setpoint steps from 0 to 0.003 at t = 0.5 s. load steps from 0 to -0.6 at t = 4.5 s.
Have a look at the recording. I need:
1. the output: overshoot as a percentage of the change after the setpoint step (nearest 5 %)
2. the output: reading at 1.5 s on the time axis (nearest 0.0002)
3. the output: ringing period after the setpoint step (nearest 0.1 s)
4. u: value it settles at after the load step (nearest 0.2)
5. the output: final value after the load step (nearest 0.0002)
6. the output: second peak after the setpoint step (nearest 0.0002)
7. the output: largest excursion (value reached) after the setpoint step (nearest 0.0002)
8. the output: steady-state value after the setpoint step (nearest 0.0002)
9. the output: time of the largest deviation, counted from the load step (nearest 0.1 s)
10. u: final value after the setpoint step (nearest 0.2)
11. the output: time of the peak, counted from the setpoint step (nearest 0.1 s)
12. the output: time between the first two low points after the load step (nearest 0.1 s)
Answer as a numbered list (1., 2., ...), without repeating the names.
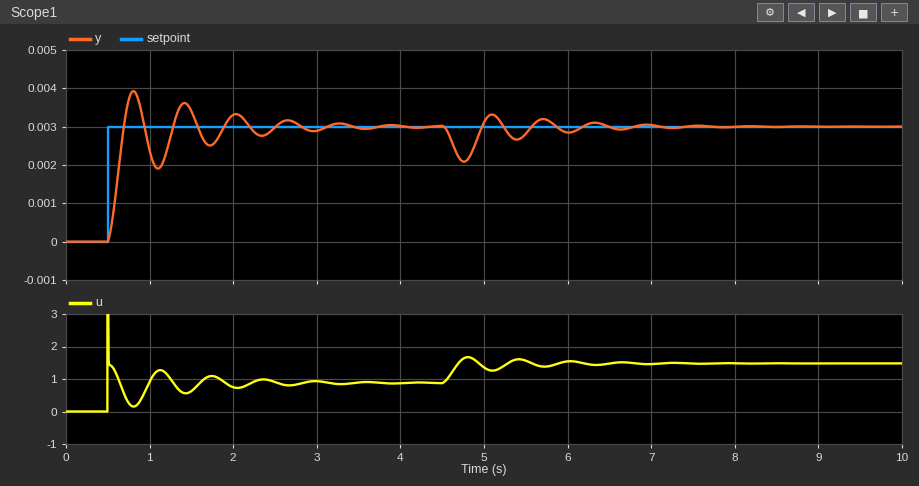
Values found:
1. 30 %
2. 0.0034
3. 0.6 s
4. 1.4
5. 0.0030
6. 0.0036
7. 0.0040
8. 0.0030
9. 0.3 s
10. 0.8
11. 0.3 s
12. 0.6 s
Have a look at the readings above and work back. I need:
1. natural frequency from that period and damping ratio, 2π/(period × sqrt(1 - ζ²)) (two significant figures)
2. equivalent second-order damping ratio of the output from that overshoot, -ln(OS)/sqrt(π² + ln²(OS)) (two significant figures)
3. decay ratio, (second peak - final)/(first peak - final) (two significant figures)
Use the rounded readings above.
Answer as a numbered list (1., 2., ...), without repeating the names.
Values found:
1. 11 rad/s
2. 0.36
3. 0.60
